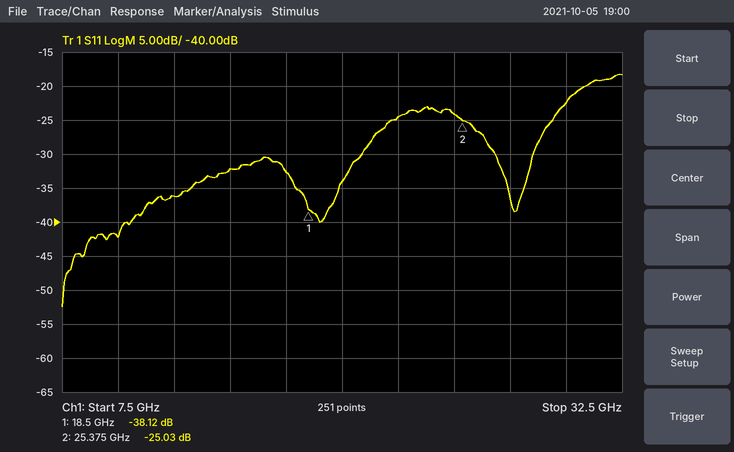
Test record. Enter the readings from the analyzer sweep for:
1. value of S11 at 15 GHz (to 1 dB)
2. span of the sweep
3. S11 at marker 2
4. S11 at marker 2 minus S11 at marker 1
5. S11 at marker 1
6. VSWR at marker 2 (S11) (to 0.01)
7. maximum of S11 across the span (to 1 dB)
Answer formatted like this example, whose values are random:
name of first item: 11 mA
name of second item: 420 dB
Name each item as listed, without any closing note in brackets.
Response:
value of S11 at 15 GHz: -32 dB
span of the sweep: 25 GHz
S11 at marker 2: -25.03 dB
S11 at marker 2 minus S11 at marker 1: 13.09 dB
S11 at marker 1: -38.12 dB
VSWR at marker 2 (S11): 1.12
maximum of S11 across the span: -18 dB
